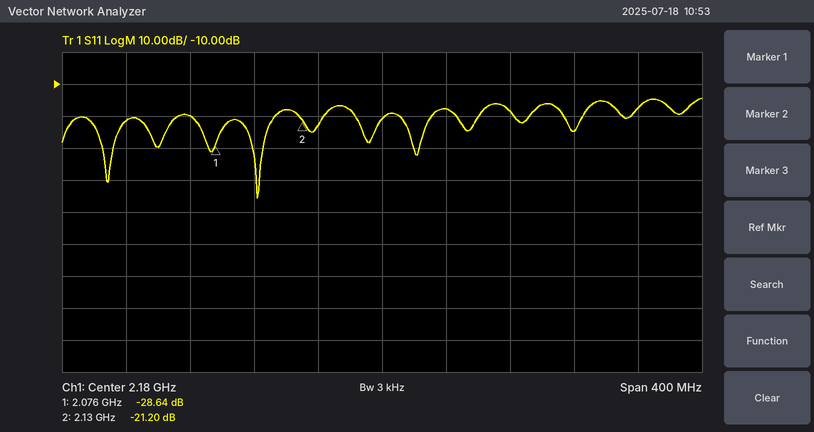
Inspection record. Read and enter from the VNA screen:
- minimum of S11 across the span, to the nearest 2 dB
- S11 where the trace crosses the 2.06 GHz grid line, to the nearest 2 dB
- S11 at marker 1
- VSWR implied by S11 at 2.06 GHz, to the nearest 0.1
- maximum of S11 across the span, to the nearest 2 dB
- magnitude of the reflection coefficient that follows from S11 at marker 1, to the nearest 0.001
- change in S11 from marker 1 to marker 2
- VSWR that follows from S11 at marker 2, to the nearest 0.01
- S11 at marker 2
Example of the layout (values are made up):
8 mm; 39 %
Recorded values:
-46 dB; -20 dB; -28.64 dB; 1.2; -14 dB; 0.037; 7.44 dB; 1.19; -21.20 dB
